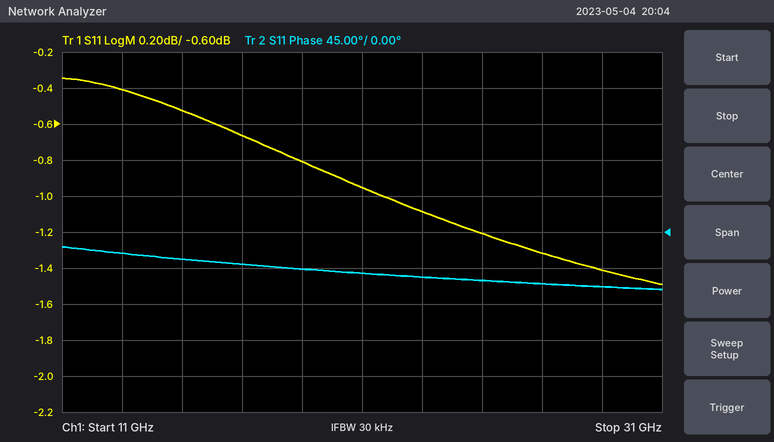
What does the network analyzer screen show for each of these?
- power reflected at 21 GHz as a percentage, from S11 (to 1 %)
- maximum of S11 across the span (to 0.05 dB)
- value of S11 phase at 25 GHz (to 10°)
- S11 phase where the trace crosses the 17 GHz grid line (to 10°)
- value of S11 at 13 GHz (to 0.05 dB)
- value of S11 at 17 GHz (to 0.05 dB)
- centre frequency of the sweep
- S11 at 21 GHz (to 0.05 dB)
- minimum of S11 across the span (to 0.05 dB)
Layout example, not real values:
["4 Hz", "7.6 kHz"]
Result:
["80 %", "-0.35 dB", "-60°", "-40°", "-0.40 dB", "-0.65 dB", "21 GHz", "-0.95 dB", "-1.50 dB"]
